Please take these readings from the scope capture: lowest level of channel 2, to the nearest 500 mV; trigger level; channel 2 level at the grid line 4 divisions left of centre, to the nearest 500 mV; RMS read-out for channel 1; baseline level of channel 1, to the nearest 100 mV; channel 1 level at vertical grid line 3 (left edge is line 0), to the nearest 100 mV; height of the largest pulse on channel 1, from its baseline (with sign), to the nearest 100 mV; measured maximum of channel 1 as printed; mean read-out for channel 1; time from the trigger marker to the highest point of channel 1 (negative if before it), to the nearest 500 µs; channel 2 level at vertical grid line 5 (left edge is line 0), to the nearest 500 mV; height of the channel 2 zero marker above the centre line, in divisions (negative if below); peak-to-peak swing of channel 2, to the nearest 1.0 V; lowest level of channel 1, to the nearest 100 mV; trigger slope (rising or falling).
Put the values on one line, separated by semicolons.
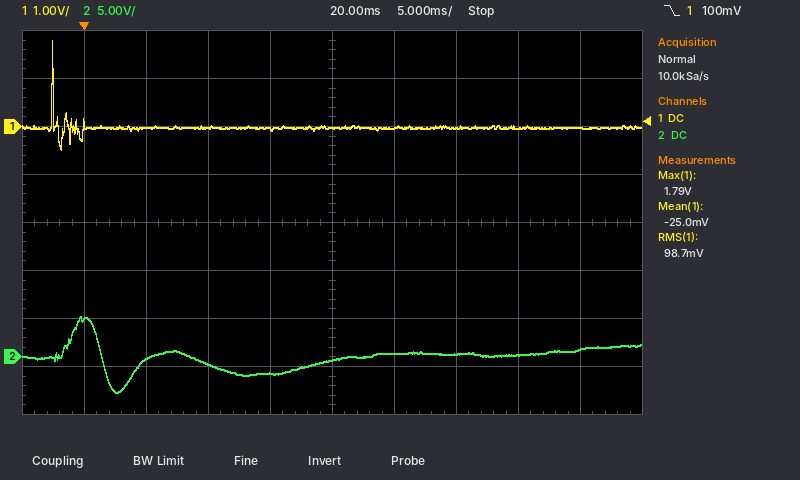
-3.5 V; 100 mV; 4.0 V; 98.7 mV; 0.0 V; 0.0 V; +1.8 V; 1.79 V; -25.0 mV; -2.5 ms; -500 mV; -2.8 div; 8.0 V; -500 mV; falling
